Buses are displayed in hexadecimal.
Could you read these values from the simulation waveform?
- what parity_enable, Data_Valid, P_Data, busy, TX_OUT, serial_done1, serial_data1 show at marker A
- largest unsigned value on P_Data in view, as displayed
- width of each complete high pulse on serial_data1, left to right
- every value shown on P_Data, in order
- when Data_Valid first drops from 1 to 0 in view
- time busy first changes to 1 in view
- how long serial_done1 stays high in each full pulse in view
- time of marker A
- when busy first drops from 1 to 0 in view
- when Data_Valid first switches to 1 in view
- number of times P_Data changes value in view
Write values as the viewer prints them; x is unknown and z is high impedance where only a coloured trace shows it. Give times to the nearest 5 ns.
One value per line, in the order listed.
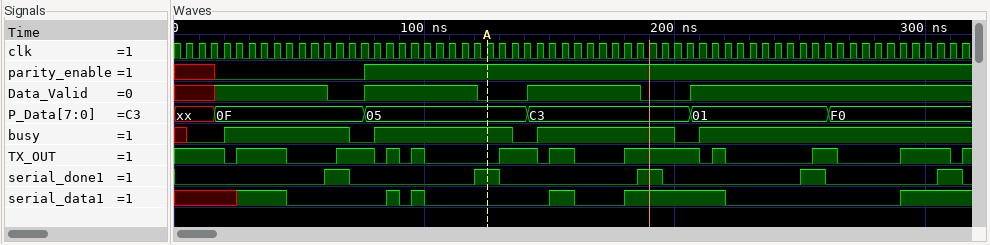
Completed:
parity_enable=1, Data_Valid=0, P_Data=05, busy=1, TX_OUT=0, serial_done1=1, serial_data1=0
F0
5 ns, 5 ns, 10 ns, 40 ns
xx, 0F, 05, C3, 01, F0
60 ns
20 ns
10 ns, 10 ns, 10 ns, 10 ns, 10 ns
125 ns
70 ns
15 ns
5
